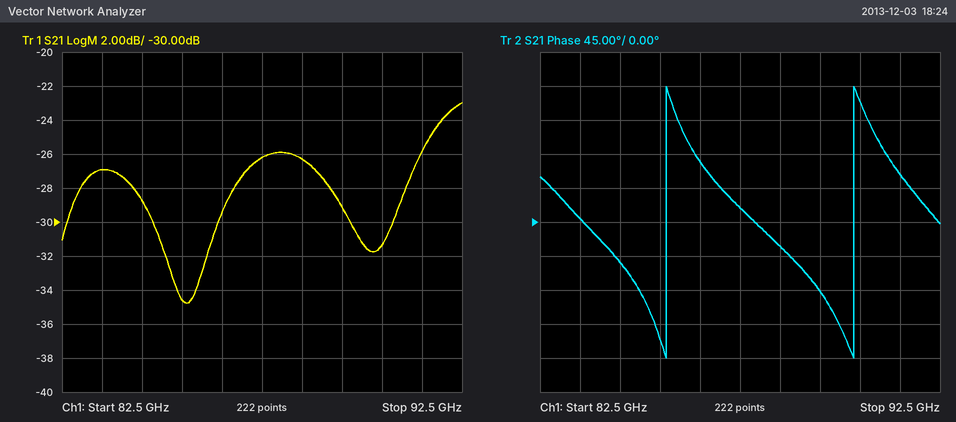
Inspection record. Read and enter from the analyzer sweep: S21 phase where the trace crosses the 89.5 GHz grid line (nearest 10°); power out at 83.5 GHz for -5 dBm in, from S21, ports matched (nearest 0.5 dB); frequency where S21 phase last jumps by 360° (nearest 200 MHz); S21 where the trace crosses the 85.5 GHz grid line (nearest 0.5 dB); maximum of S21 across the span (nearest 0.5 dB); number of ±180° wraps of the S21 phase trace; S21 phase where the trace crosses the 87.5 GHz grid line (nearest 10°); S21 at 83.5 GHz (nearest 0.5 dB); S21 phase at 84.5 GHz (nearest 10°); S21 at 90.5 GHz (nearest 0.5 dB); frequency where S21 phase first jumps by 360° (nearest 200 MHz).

-90°
-32.0 dBm
90.4 GHz
-34.5 dB
-23.0 dB
2
20°
-27.0 dB
-50°
-31.5 dB
85.6 GHz
